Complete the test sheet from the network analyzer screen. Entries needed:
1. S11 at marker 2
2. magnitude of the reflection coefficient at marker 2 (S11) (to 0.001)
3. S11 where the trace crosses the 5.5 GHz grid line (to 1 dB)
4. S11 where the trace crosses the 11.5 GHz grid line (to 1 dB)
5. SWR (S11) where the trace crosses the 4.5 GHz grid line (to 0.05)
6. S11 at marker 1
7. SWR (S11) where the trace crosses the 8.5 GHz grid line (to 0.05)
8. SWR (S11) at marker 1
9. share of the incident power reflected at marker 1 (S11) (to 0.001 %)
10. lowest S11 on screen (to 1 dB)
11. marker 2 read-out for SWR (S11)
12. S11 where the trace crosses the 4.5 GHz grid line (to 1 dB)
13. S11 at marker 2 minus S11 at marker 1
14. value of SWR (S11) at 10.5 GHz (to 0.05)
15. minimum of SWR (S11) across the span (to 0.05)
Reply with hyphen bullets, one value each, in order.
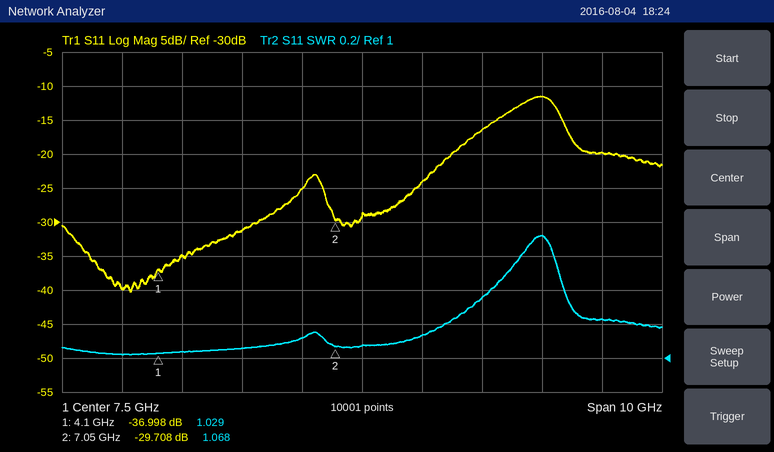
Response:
- -29.708 dB
- 0.033
- -31 dB
- -20 dB
- 1.05
- -36.998 dB
- 1.15
- 1.029
- 0.020 %
- -40 dB
- 1.068
- -35 dB
- 7.290 dB
- 1.70
- 1.00
